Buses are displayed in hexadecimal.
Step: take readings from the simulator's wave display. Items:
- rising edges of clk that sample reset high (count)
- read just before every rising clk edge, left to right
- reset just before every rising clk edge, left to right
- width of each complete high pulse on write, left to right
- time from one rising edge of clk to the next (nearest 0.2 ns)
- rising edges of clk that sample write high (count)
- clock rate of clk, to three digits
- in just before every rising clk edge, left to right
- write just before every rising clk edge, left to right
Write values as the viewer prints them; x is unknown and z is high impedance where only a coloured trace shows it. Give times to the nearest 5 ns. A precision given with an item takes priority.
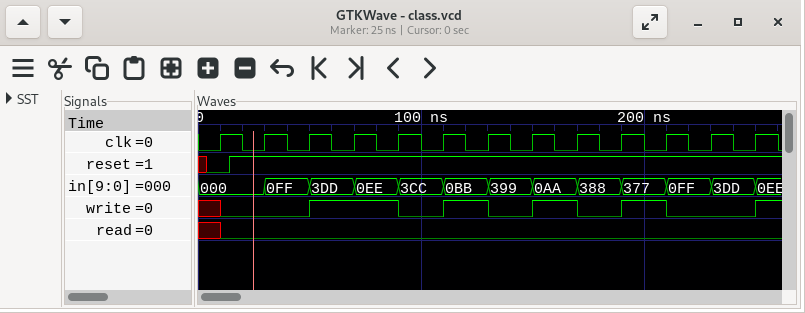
12
x 0 0 0 0 0 0 0 0 0 0 0 0
0 1 1 1 1 1 1 1 1 1 1 1 1
40 ns, 20 ns, 20 ns, 20 ns
20 ns
5
50.0 MHz
000, 000, 0FF, 3DD, 0EE, 3CC, 0BB, 399, 0AA, 388, 377, 0FF, 3DD
x 0 0 1 1 0 1 0 1 0 1 0 0
